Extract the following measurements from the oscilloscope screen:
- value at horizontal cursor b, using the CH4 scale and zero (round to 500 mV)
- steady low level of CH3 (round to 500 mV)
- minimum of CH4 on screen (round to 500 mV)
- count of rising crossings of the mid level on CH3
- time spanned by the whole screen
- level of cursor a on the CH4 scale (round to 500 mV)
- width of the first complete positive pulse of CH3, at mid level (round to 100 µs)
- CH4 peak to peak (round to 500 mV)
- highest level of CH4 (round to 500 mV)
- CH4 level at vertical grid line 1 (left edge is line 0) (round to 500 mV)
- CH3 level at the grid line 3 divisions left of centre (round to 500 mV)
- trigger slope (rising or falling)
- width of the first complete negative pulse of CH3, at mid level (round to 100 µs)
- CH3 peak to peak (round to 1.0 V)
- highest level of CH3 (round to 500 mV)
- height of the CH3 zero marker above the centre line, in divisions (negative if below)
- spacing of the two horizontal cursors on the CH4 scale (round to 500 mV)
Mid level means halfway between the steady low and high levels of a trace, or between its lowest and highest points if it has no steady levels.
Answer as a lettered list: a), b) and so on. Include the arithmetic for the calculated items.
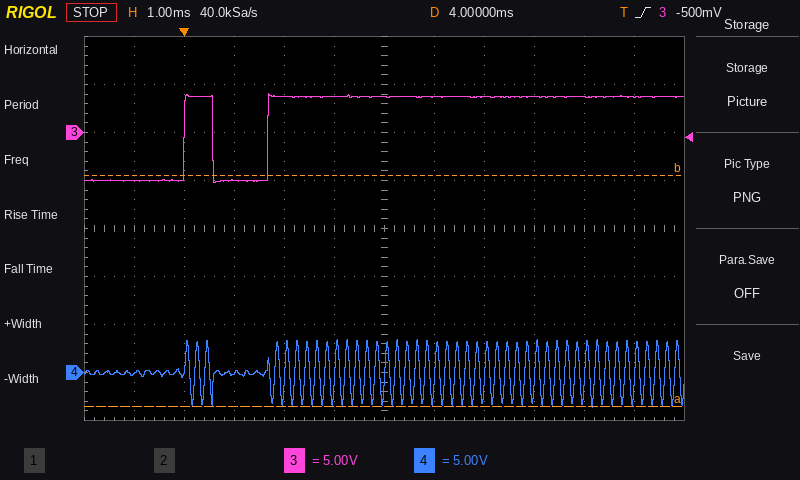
a) 20.5 V
b) -5.0 V
c) -3.5 V
d) 2
e) 12 ms
f) -3.5 V
g) 600 µs
h) 3.5 V − (-3.5 V) = 7.0 V
i) 3.5 V
j) 0.0 V
k) -5.0 V
l) rising
m) 1.1 ms
n) 9.0 V
o) 4.0 V
p) +2.0 div
q) 24.0 V
